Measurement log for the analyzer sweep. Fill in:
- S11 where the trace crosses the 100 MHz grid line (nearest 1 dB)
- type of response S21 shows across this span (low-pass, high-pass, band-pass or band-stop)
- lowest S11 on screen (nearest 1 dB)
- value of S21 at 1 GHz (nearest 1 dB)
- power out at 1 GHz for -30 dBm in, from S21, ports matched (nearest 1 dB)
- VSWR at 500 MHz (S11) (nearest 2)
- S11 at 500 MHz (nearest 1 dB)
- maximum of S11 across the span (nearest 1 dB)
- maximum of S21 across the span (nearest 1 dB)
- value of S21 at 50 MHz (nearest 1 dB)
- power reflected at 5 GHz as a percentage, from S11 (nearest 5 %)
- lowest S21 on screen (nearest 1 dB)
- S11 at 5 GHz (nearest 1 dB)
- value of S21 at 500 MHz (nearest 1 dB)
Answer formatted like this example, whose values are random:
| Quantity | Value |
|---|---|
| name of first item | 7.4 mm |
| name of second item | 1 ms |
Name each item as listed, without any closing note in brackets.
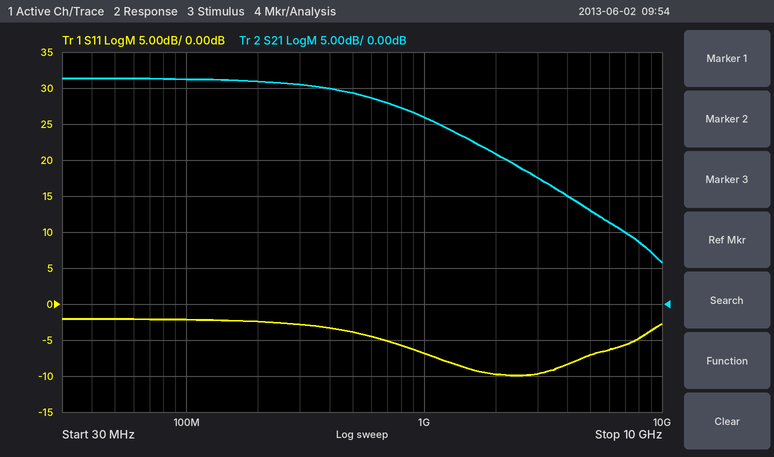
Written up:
| Quantity | Value |
|---|---|
| S11 where the trace crosses the 100 MHz grid line | -2 dB |
| type of response S21 shows across this span | low-pass |
| lowest S11 on screen | -10 dB |
| value of S21 at 1 GHz | 26 dB |
| power out at 1 GHz for -30 dBm in, from S21, ports matched | -4 dBm |
| VSWR at 500 MHz (S11) | 4 |
| S11 at 500 MHz | -4 dB |
| maximum of S11 across the span | -2 dB |
| maximum of S21 across the span | 31 dB |
| value of S21 at 50 MHz | 31 dB |
| power reflected at 5 GHz as a percentage, from S11 | 20 % |
| lowest S21 on screen | 6 dB |
| S11 at 5 GHz | -7 dB |
| value of S21 at 500 MHz | 29 dB |
